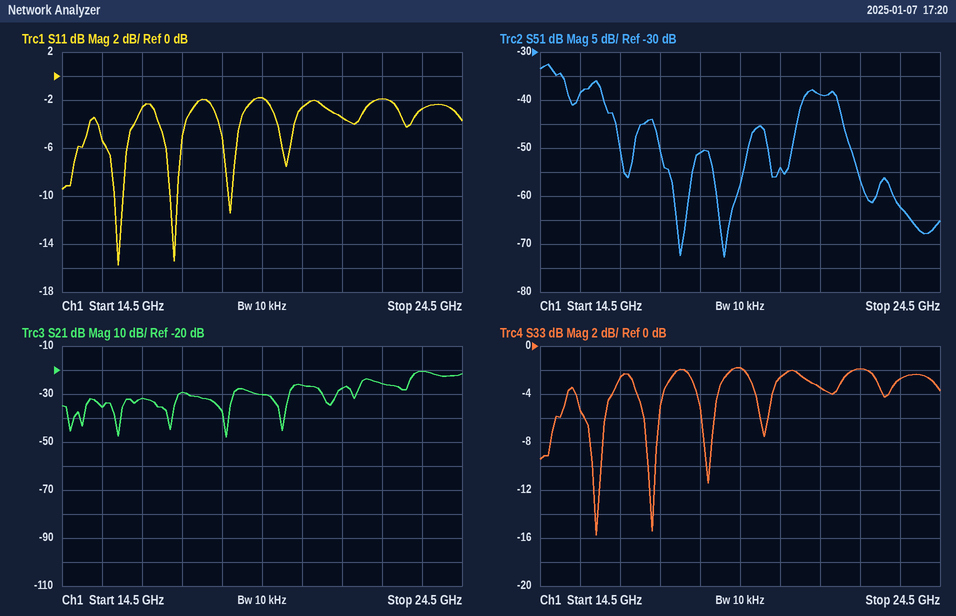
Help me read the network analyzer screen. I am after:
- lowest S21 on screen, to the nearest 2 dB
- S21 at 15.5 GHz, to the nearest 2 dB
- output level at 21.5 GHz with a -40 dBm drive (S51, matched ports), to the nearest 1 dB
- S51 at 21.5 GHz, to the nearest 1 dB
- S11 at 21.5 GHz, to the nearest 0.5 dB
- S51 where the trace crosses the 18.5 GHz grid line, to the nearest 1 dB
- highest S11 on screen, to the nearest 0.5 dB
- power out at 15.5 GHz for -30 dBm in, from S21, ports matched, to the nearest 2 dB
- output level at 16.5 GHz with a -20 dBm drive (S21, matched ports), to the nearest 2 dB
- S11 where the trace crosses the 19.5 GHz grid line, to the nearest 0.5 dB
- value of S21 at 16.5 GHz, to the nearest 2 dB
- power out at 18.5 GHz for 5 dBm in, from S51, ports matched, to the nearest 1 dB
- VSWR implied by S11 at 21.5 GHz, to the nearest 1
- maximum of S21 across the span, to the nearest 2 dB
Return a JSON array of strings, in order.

["-48 dB", "-36 dB", "-79 dBm", "-39 dB", "-3.5 dB", "-51 dB", "-2.0 dB", "-66 dBm", "-52 dBm", "-2.0 dB", "-32 dB", "-46 dBm", "5", "-20 dB"]
